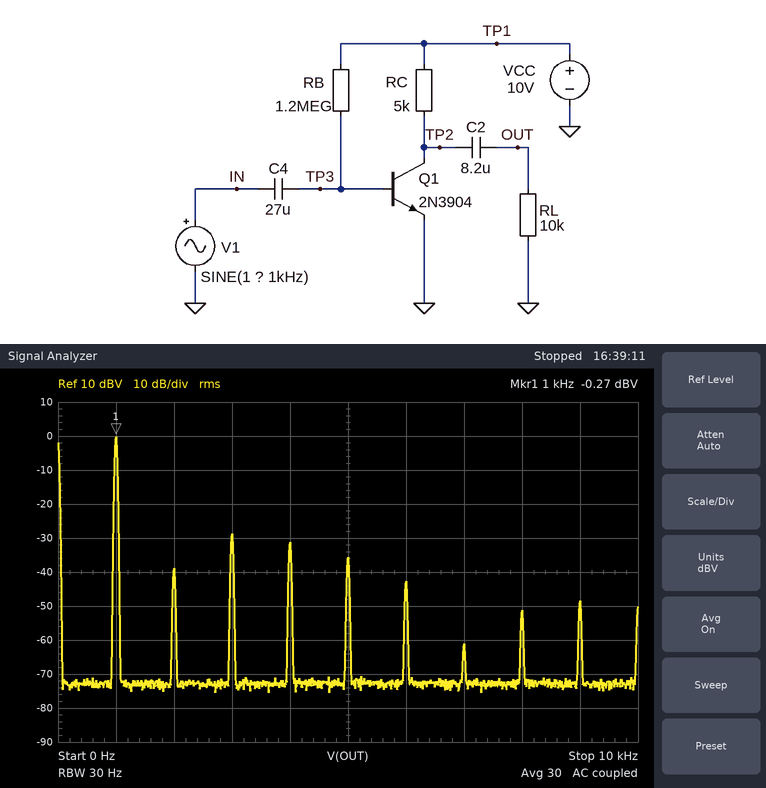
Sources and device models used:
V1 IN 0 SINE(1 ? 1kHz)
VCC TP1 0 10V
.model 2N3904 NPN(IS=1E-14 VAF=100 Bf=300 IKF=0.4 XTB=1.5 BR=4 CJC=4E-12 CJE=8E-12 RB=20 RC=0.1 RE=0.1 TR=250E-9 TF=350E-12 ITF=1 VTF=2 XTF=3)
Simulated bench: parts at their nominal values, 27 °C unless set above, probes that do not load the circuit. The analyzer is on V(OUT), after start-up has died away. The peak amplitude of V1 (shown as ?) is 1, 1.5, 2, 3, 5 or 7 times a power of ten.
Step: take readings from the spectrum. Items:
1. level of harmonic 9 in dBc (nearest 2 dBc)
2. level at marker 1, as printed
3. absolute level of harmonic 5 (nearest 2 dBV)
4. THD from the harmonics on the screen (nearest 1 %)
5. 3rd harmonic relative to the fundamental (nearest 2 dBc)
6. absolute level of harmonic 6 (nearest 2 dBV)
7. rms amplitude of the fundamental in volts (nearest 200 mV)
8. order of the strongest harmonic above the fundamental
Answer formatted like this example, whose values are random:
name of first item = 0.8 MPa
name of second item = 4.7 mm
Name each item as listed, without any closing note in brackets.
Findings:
level of harmonic 9 in dBc = -48 dBc
level at marker 1, as printed = -0.27 dBV
absolute level of harmonic 5 = -36 dBV
THD from the harmonics on the screen = 5 %
3rd harmonic relative to the fundamental = -28 dBc
absolute level of harmonic 6 = -42 dBV
rms amplitude of the fundamental in volts = 1.0 V
order of the strongest harmonic above the fundamental = 3
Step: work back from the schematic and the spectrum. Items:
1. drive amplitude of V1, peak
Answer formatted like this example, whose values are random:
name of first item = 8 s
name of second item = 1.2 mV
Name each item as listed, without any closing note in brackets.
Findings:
drive amplitude of V1, peak = 7 mV
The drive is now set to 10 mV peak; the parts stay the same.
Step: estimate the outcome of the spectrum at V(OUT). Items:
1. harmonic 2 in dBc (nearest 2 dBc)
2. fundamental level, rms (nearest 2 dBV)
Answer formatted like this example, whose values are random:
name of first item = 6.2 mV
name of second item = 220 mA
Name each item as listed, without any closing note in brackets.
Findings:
harmonic 2 in dBc = -28 dBc
fundamental level, rms = 2 dBV
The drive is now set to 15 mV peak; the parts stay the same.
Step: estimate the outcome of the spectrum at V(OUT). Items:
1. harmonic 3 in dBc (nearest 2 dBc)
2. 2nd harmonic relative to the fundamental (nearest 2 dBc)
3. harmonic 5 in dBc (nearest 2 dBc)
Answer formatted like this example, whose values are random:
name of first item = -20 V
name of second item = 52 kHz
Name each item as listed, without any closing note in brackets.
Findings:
harmonic 3 in dBc = -32 dBc
2nd harmonic relative to the fundamental = -20 dBc
harmonic 5 in dBc = -34 dBc
